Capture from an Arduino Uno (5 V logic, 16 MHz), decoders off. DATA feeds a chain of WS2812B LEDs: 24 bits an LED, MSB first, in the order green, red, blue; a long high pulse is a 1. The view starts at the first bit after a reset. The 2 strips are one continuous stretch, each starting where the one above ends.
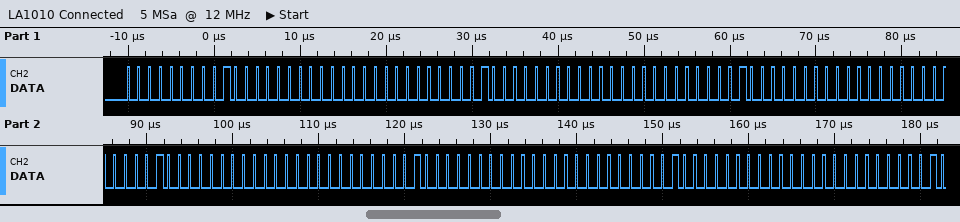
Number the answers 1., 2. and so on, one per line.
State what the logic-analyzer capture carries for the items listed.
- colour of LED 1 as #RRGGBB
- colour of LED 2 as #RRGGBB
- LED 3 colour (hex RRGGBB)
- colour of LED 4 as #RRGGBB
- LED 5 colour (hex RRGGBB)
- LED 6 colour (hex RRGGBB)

1. #400000
2. #400000
3. #400000
4. #400000
5. #400000
6. #400000
